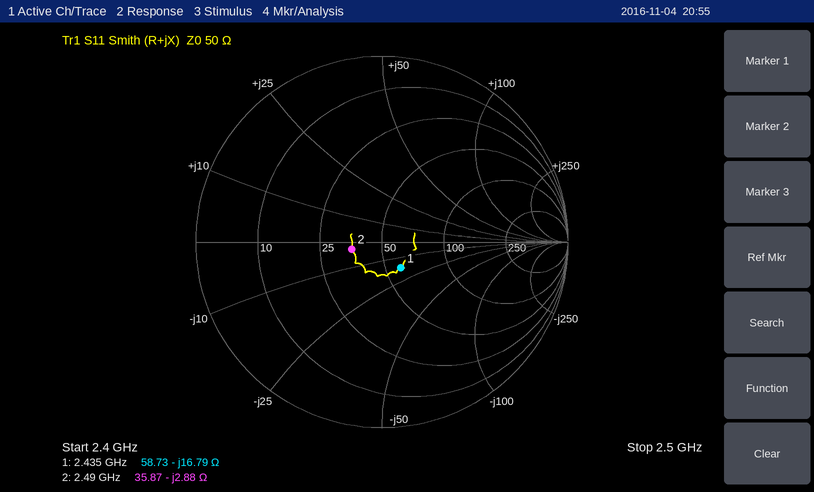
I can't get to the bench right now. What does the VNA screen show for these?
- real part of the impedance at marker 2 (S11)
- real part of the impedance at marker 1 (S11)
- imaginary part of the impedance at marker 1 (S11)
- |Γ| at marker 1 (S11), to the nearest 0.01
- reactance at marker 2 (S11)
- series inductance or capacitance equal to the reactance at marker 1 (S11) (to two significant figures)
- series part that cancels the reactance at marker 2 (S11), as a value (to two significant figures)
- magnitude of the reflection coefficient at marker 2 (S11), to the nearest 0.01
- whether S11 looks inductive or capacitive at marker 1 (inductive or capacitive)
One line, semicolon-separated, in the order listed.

35.87 Ω; 58.73 Ω; -16.79 Ω; 0.17; -2.88 Ω; 3.9 pF; 180 pH; 0.17; capacitive
